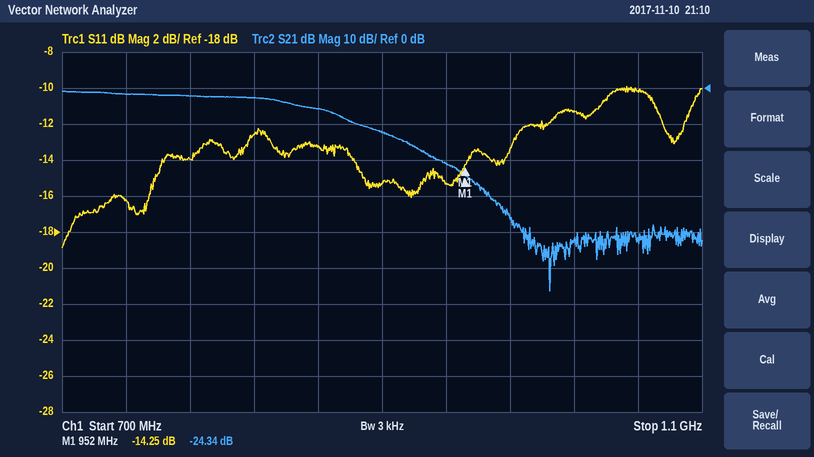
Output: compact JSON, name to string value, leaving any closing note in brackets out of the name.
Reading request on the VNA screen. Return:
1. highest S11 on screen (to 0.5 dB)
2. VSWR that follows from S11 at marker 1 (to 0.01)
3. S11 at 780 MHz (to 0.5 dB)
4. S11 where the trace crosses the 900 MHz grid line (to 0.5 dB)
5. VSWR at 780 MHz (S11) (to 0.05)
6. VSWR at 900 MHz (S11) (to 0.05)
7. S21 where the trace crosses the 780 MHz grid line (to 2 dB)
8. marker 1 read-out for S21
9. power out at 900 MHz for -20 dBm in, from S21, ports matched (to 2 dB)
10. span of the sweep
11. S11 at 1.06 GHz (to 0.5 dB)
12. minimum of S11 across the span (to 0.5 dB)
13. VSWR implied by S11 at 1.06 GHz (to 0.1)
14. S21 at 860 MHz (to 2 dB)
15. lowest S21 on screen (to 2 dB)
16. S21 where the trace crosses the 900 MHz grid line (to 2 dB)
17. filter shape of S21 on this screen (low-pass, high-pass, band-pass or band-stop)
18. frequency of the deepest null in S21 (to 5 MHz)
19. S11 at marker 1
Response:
{"highest S11 on screen": "-10.0 dB", "VSWR that follows from S11 at marker 1": "1.48", "S11 at 780 MHz": "-14.0 dB", "S11 where the trace crosses the 900 MHz grid line": "-15.5 dB", "VSWR at 780 MHz (S11)": "1.50", "VSWR at 900 MHz (S11)": "1.40", "S21 where the trace crosses the 780 MHz grid line": "-2 dB", "marker 1 read-out for S21": "-24.34 dB", "power out at 900 MHz for -20 dBm in, from S21, ports matched": "-32 dBm", "span of the sweep": "400 MHz", "S11 at 1.06 GHz": "-10.0 dB", "minimum of S11 across the span": "-19.0 dB", "VSWR implied by S11 at 1.06 GHz": "1.9", "S21 at 860 MHz": "-6 dB", "lowest S21 on screen": "-56 dB", "S21 where the trace crosses the 900 MHz grid line": "-12 dB", "filter shape of S21 on this screen": "low-pass", "frequency of the deepest null in S21": "1.005 GHz", "S11 at marker 1": "-14.25 dB"}
